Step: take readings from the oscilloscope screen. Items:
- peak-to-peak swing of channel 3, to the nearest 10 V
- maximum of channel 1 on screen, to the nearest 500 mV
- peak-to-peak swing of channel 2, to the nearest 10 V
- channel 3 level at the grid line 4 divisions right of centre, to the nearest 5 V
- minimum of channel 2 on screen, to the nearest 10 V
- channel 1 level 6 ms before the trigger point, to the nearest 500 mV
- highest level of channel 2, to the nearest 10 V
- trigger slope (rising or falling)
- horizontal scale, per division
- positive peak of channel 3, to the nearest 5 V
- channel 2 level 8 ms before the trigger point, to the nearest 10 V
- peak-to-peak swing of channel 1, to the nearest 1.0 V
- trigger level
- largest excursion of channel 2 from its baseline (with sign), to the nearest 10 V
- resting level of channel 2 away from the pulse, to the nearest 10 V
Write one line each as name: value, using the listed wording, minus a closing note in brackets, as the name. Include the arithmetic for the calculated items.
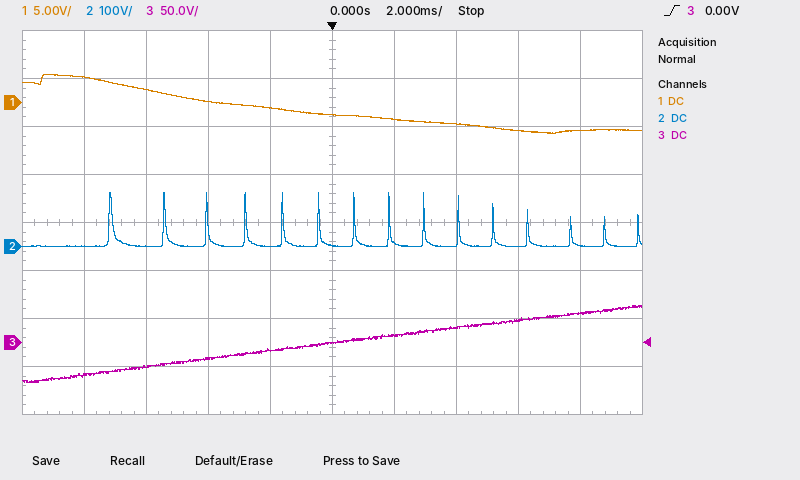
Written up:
peak-to-peak swing of channel 3, to the nearest 10 V: 80 V
maximum of channel 1 on screen, to the nearest 500 mV: 3.0 V
peak-to-peak swing of channel 2, to the nearest 10 V: 110 V − (0 V) = 110 V
channel 3 level at the grid line 4 divisions right of centre, to the nearest 5 V: 30 V
minimum of channel 2 on screen, to the nearest 10 V: 0 V
channel 1 level 6 ms before the trigger point, to the nearest 500 mV: 1.5 V
highest level of channel 2, to the nearest 10 V: 110 V
trigger slope: rising
horizontal scale, per division: 2 ms
positive peak of channel 3, to the nearest 5 V: 40 V
channel 2 level 8 ms before the trigger point, to the nearest 10 V: 0 V
peak-to-peak swing of channel 1, to the nearest 1.0 V: 6.0 V
trigger level: 0.00 V
largest excursion of channel 2 from its baseline (with sign), to the nearest 10 V: 110 V − (0 V) = +110 V
resting level of channel 2 away from the pulse, to the nearest 10 V: 0 V
